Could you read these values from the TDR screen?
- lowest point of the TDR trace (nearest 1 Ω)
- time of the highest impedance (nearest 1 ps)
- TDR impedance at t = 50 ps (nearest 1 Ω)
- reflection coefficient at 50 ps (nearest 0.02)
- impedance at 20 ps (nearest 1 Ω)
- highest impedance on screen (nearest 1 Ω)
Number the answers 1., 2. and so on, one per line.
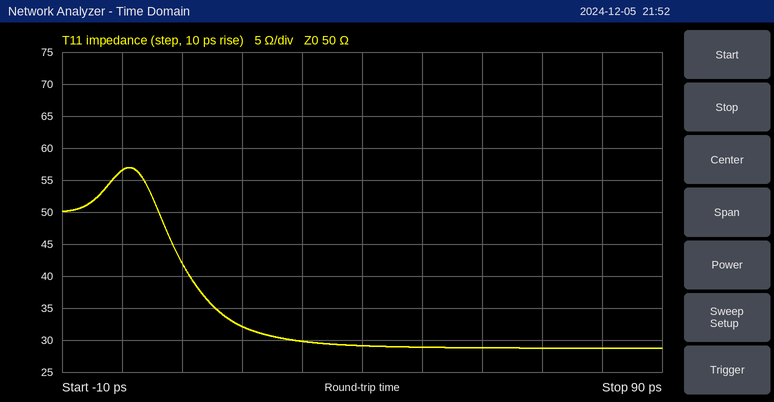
1. 29 Ω
2. 1 ps
3. 29 Ω
4. -0.26
5. 32 Ω
6. 57 Ω
